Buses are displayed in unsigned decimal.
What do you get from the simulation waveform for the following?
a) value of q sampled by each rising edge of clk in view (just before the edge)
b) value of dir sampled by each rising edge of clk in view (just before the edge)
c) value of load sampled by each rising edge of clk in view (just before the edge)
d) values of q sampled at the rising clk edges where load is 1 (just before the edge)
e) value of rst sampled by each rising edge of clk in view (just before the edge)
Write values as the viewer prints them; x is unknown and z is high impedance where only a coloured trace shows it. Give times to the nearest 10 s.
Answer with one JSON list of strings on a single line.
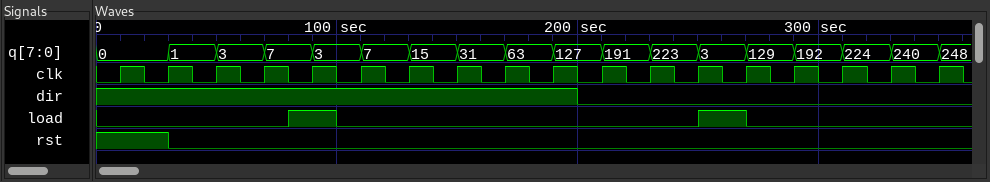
["0, 0, 1, 3, 7, 3, 7, 15, 31, 63, 127, 191, 223, 3, 129, 192, 224, 240", "1 1 1 1 1 1 1 1 1 1 0 0 0 0 0 0 0 0", "0 0 0 0 1 0 0 0 0 0 0 0 0 1 0 0 0 0", "7, 3", "1 1 0 0 0 0 0 0 0 0 0 0 0 0 0 0 0 0"]
